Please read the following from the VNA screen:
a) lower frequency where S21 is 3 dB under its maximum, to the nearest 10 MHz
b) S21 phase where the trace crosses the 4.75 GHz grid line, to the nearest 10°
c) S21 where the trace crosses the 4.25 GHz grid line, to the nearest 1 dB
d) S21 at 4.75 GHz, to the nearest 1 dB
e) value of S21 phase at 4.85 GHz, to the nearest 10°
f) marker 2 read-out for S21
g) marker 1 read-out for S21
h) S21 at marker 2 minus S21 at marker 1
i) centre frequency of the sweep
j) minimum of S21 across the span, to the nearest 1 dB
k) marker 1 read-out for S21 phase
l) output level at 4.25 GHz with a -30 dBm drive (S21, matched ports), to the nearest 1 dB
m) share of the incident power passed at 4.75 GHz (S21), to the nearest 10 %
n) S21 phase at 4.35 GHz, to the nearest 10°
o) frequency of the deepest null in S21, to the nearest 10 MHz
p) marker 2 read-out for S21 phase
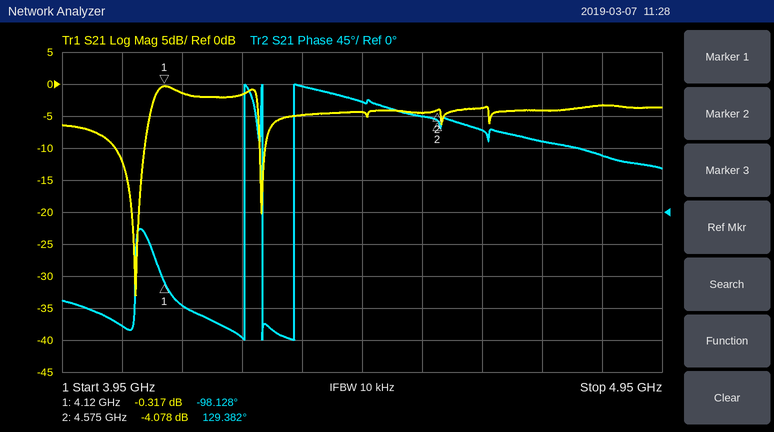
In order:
4.10 GHz
100°
-2 dB
-4 dB
80°
-4.078 dB
-0.317 dB
-3.761 dB
4.45 GHz
-33 dB
-98.128°
-32 dBm
40 %
180°
4.07 GHz
129.382°
